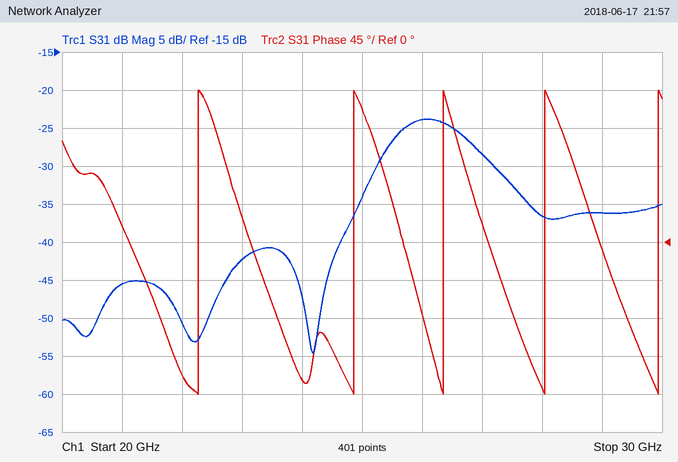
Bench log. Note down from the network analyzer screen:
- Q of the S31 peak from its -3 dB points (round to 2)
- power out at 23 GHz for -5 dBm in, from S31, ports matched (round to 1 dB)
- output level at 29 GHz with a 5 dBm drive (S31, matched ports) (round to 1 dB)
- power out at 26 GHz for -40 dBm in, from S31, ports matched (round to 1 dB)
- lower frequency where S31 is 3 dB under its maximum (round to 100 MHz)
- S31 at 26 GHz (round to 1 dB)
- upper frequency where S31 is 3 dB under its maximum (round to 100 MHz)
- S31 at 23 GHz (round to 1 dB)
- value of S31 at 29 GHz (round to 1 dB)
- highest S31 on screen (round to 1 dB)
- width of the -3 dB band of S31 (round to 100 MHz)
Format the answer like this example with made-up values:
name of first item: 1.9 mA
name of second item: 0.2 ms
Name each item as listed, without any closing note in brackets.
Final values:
Q of the S31 peak from its -3 dB points: 20
power out at 23 GHz for -5 dBm in, from S31, ports matched: -47 dBm
output level at 29 GHz with a 5 dBm drive (S31, matched ports): -31 dBm
power out at 26 GHz for -40 dBm in, from S31, ports matched: -64 dBm
lower frequency where S31 is 3 dB under its maximum: 25.5 GHz
S31 at 26 GHz: -24 dB
upper frequency where S31 is 3 dB under its maximum: 26.8 GHz
S31 at 23 GHz: -42 dB
value of S31 at 29 GHz: -36 dB
highest S31 on screen: -24 dB
width of the -3 dB band of S31: 1.3 GHz
